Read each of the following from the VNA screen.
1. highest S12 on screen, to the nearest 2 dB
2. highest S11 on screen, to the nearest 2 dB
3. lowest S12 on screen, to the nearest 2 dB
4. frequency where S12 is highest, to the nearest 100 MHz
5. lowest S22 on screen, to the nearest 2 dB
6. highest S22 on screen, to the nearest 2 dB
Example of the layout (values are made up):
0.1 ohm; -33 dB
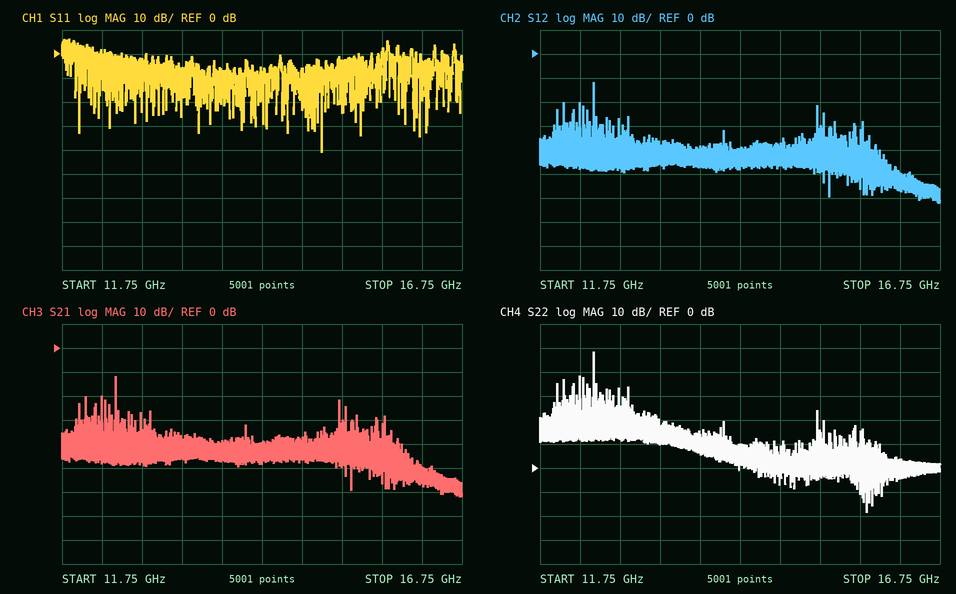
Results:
-12 dB; 6 dB; -62 dB; 12.4 GHz; -18 dB; 48 dB
